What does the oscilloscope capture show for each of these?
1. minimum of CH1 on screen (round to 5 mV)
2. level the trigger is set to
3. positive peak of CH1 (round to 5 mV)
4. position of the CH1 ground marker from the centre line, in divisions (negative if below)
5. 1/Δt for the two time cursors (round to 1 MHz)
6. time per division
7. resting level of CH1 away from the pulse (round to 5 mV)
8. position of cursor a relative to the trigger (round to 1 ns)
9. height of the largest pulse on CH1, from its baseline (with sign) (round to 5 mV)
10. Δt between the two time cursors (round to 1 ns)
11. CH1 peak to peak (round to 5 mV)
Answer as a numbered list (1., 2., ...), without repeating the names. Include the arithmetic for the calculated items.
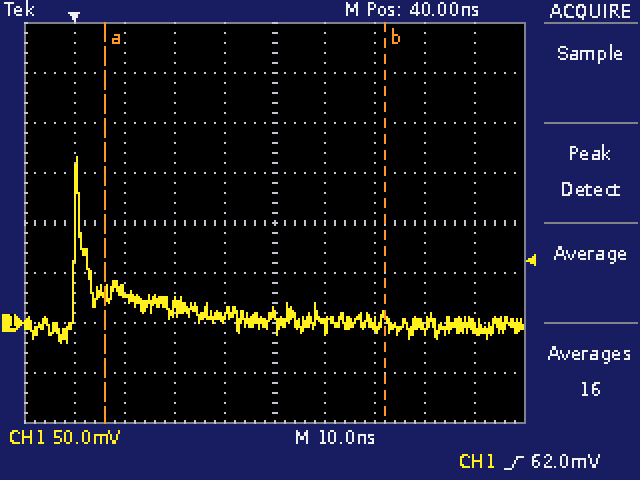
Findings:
1. -20 mV
2. 62.0 mV
3. 165 mV
4. -2.0 div
5. 1 / 56 ns ≈ 18 MHz
6. 10 ns
7. 0 mV
8. +6 ns
9. 165 mV − (0 mV) = +165 mV
10. 56 ns
11. 165 mV − (-20 mV) = 185 mV
